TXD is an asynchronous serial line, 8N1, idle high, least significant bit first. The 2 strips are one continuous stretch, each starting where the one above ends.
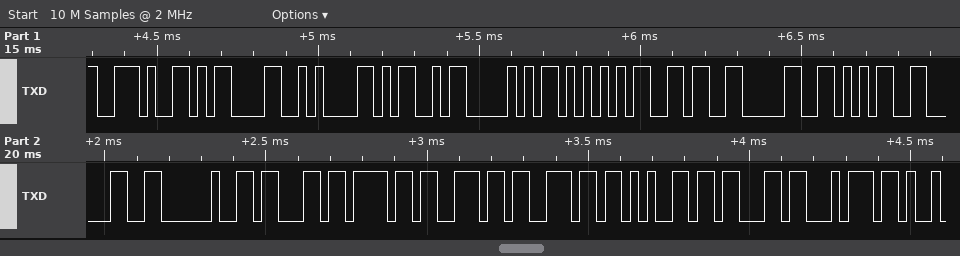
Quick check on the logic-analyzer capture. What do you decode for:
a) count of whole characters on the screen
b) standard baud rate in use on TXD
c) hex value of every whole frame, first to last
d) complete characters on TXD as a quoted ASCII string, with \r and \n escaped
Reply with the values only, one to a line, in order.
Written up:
18
38400 baud
2E 0D 0A 4D 50 55 36 30 35 30 20 63 6F 6E 6E 65 63 74
".\r\nMPU6050 connect"
